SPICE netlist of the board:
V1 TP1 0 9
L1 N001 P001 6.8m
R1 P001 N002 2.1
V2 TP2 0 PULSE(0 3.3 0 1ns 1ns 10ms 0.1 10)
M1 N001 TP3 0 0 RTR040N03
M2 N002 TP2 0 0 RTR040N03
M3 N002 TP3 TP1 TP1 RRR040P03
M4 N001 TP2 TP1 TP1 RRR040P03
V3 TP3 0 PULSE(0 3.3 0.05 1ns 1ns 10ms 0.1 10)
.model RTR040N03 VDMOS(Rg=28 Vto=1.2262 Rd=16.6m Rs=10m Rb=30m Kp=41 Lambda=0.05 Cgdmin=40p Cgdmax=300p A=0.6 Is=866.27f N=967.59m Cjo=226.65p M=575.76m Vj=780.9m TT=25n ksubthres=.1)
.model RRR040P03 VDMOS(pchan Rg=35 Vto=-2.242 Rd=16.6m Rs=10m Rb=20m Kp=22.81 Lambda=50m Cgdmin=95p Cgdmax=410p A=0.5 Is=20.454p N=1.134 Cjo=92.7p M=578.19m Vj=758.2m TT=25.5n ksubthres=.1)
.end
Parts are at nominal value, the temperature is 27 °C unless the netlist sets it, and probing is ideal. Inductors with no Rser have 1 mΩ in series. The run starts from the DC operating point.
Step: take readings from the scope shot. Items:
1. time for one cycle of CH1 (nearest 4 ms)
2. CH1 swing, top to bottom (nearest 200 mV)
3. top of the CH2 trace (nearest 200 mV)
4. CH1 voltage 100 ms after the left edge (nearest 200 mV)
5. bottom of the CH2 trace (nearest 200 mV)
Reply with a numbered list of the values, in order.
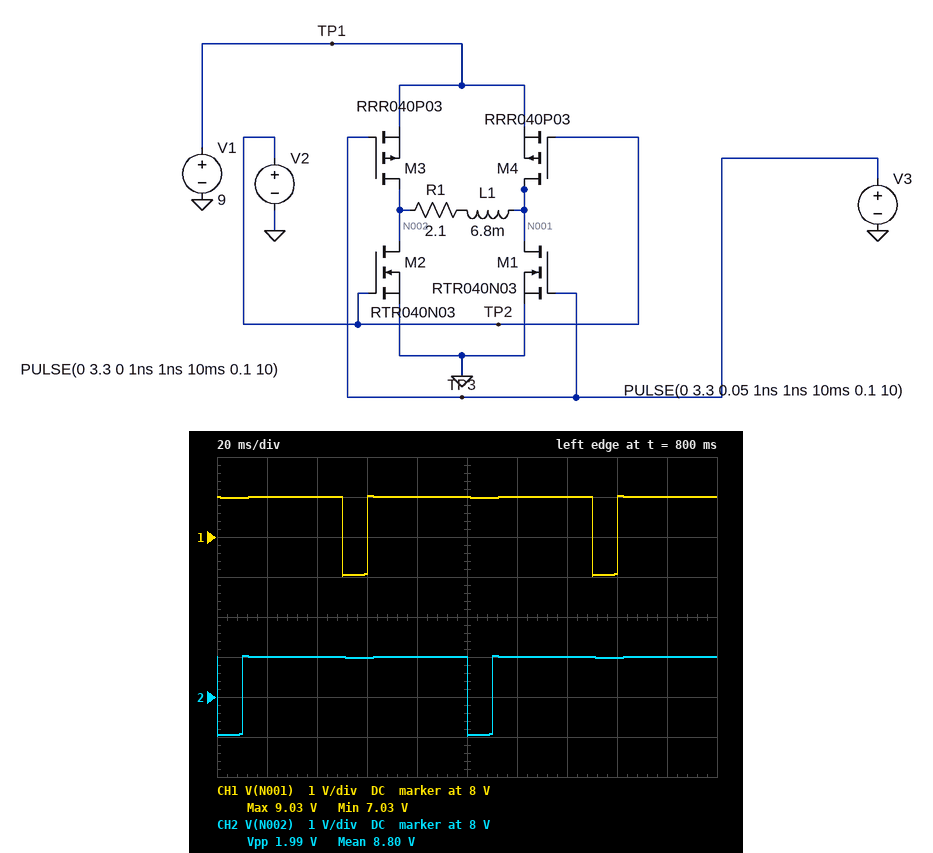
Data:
1. 100 ms
2. 2.0 V
3. 9.0 V
4. 9.0 V
5. 7.0 V
